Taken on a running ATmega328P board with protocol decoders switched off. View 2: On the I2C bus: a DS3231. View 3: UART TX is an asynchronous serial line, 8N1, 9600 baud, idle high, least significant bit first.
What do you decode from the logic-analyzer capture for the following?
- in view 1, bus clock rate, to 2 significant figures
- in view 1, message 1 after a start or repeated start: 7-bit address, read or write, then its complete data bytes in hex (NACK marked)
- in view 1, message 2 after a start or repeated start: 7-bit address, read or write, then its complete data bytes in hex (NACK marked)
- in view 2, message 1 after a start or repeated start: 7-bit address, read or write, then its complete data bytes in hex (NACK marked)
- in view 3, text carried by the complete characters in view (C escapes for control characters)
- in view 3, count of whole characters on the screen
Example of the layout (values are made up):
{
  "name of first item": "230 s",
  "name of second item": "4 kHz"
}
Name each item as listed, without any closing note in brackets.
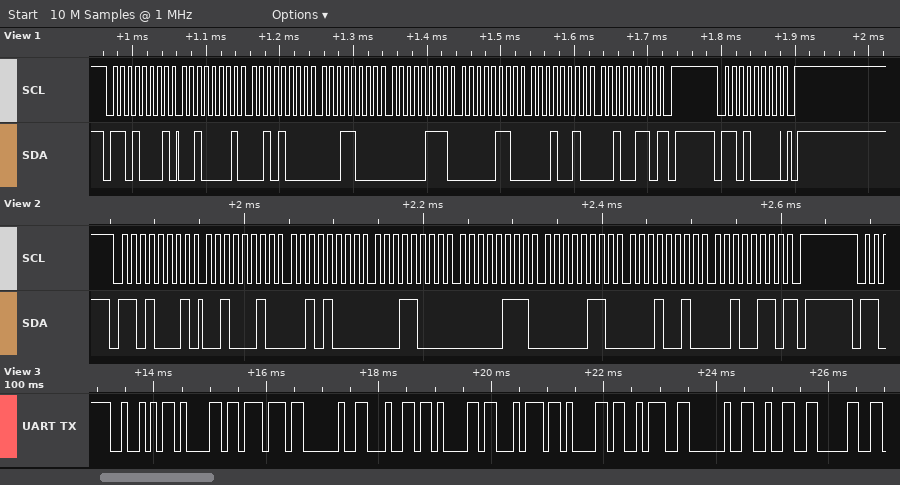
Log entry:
{
  "in view 1, bus clock rate, to 2 significant figures": "100 kHz",
  "in view 1, message 1 after a start or repeated start: 7-bit address, read or write, then its complete data bytes in hex": "0x68 read: 21 28 18 07 06 12 26 NACK",
  "in view 1, message 2 after a start or repeated start: 7-bit address, read or write, then its complete data bytes in hex": "0x68 write",
  "in view 2, message 1 after a start or repeated start: 7-bit address, read or write, then its complete data bytes in hex": "0x68 read: 22 28 18 07 06 12 26 NACK",
  "in view 3, text carried by the complete characters in view": "\"Raw data: 20\"",
  "in view 3, count of whole characters on the screen": "12"
}
